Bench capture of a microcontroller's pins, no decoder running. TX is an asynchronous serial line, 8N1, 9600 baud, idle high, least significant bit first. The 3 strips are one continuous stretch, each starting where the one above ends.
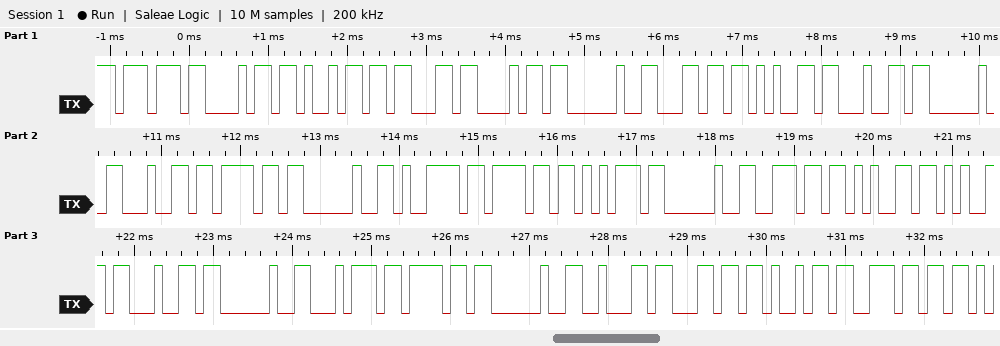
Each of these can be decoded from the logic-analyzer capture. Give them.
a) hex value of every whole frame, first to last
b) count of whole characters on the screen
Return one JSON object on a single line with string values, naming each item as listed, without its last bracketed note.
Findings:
{"hex value of every whole frame, first to last": "77 68 69 63 68 20 6C 65 64 20 64 6F 20 79 6F 75 20 6E 65 65 64 20 74 6F 20 62 6C 69 6E", "count of whole characters on the screen": "29"}
